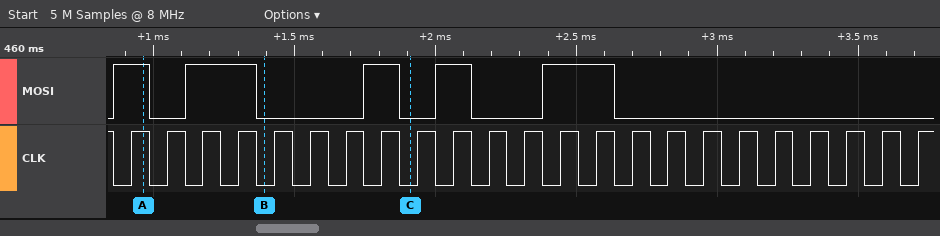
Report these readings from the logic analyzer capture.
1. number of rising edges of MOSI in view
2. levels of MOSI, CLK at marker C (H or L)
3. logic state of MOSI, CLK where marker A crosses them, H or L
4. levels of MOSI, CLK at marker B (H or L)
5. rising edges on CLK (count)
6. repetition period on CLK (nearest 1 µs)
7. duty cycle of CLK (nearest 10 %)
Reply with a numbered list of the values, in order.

1. 5
2. MOSI=L, CLK=L
3. MOSI=H, CLK=H
4. MOSI=L, CLK=L
5. 23
6. 127 µs
7. 50 %
